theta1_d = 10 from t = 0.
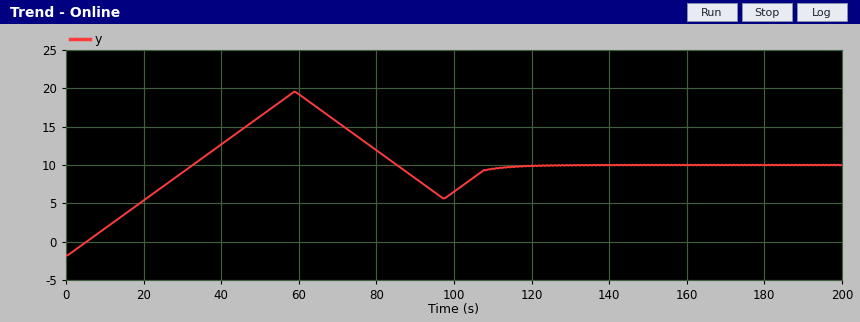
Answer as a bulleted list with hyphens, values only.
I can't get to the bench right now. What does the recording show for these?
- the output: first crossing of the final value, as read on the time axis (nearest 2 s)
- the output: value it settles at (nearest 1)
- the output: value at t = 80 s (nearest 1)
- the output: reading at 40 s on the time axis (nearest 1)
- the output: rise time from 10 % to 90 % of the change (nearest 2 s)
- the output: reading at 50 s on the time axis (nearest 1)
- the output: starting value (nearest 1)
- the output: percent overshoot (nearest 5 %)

- 32 s
- 10
- 12
- 13
- 26 s
- 16
- -2
- 80 %
